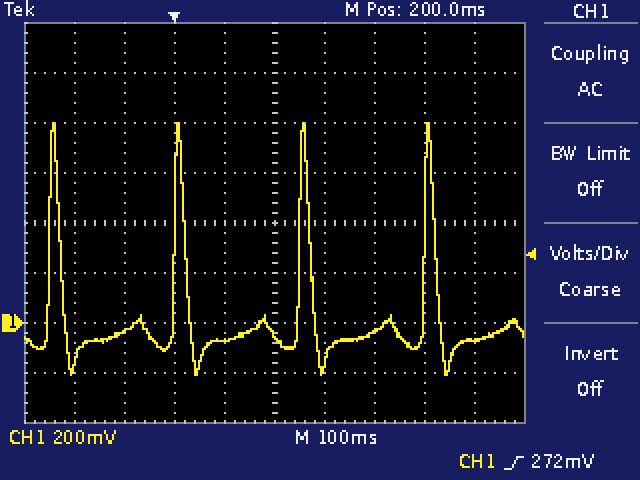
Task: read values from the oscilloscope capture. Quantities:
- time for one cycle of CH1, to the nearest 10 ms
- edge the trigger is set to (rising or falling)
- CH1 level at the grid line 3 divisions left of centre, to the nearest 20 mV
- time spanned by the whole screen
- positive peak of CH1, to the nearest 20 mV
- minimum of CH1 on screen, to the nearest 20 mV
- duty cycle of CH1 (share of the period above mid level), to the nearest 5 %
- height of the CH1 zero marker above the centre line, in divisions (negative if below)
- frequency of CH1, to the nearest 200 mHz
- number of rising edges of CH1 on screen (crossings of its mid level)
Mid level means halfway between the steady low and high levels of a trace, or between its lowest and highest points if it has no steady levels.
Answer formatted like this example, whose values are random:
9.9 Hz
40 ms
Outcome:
250 ms
rising
-40 mV
1 s
800 mV
-200 mV
10 %
-2.0 div
4.0 Hz
4
